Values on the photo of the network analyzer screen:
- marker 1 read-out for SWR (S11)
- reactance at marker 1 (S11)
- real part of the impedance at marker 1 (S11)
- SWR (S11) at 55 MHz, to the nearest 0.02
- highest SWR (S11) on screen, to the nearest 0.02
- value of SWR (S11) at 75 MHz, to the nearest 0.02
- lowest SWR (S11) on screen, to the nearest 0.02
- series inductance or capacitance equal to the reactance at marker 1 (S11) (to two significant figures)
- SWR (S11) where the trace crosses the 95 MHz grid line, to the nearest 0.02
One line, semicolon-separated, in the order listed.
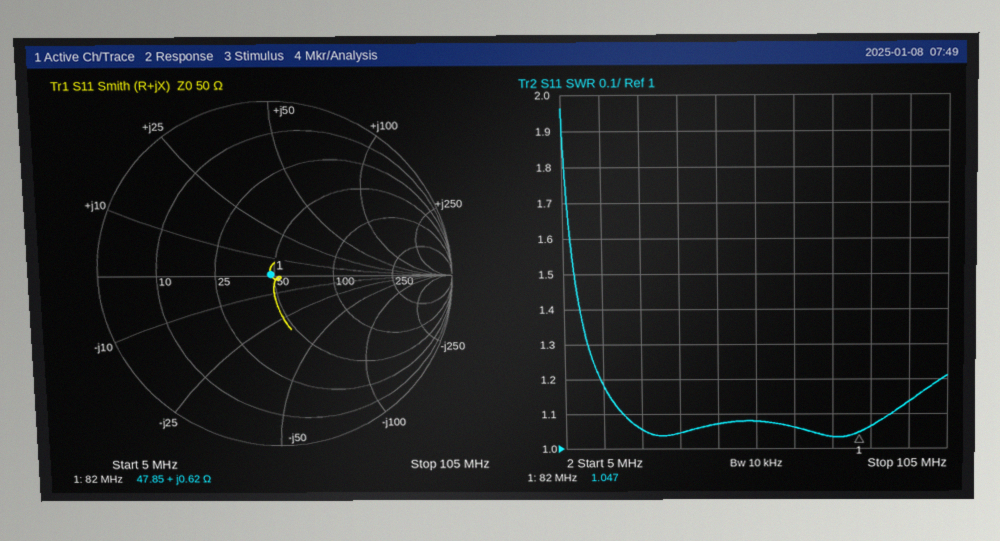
1.047; +0.62 Ω; 47.85 Ω; 1.08; 1.96; 1.04; 1.04; 1.2 nH; 1.14
